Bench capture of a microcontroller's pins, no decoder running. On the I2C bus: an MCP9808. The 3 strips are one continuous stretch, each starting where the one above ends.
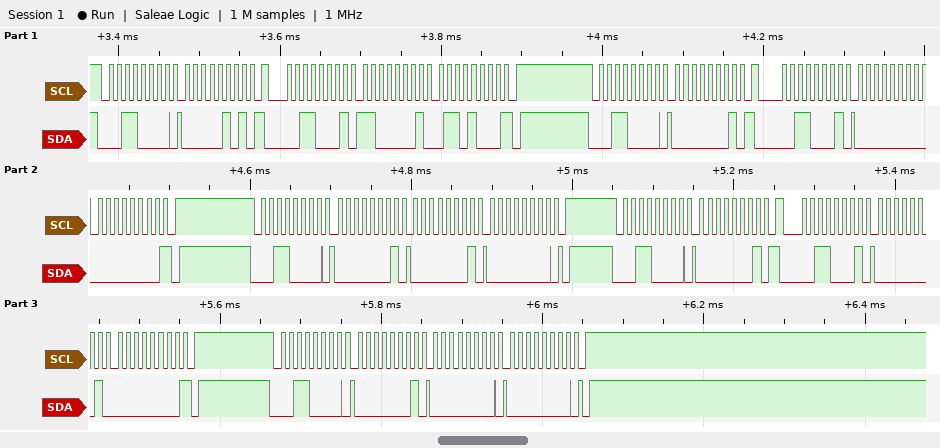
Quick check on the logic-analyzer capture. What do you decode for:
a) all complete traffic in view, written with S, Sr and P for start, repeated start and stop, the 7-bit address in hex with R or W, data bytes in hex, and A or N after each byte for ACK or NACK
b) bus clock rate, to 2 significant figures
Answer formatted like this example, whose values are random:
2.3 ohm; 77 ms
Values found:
S 18W A 05 A Sr 18R A C1 A 68 N P S 18W A 01 A Sr 18R A 00 A 00 N P S 18W A 01 A 01 A 00 A P S 18W A 01 A Sr 18R A 01 A 00 N P S 18W A 01 A 00 A 00 A P; 100 kHz
